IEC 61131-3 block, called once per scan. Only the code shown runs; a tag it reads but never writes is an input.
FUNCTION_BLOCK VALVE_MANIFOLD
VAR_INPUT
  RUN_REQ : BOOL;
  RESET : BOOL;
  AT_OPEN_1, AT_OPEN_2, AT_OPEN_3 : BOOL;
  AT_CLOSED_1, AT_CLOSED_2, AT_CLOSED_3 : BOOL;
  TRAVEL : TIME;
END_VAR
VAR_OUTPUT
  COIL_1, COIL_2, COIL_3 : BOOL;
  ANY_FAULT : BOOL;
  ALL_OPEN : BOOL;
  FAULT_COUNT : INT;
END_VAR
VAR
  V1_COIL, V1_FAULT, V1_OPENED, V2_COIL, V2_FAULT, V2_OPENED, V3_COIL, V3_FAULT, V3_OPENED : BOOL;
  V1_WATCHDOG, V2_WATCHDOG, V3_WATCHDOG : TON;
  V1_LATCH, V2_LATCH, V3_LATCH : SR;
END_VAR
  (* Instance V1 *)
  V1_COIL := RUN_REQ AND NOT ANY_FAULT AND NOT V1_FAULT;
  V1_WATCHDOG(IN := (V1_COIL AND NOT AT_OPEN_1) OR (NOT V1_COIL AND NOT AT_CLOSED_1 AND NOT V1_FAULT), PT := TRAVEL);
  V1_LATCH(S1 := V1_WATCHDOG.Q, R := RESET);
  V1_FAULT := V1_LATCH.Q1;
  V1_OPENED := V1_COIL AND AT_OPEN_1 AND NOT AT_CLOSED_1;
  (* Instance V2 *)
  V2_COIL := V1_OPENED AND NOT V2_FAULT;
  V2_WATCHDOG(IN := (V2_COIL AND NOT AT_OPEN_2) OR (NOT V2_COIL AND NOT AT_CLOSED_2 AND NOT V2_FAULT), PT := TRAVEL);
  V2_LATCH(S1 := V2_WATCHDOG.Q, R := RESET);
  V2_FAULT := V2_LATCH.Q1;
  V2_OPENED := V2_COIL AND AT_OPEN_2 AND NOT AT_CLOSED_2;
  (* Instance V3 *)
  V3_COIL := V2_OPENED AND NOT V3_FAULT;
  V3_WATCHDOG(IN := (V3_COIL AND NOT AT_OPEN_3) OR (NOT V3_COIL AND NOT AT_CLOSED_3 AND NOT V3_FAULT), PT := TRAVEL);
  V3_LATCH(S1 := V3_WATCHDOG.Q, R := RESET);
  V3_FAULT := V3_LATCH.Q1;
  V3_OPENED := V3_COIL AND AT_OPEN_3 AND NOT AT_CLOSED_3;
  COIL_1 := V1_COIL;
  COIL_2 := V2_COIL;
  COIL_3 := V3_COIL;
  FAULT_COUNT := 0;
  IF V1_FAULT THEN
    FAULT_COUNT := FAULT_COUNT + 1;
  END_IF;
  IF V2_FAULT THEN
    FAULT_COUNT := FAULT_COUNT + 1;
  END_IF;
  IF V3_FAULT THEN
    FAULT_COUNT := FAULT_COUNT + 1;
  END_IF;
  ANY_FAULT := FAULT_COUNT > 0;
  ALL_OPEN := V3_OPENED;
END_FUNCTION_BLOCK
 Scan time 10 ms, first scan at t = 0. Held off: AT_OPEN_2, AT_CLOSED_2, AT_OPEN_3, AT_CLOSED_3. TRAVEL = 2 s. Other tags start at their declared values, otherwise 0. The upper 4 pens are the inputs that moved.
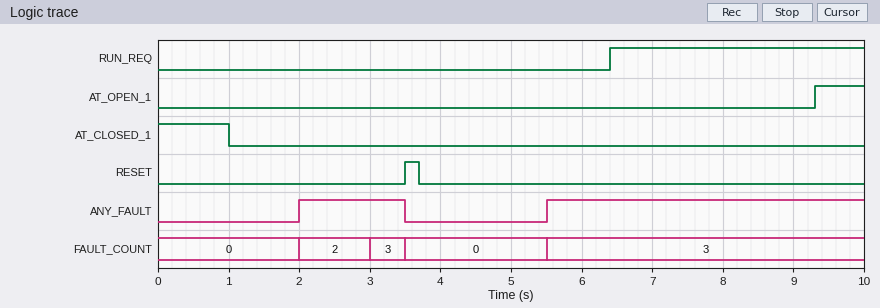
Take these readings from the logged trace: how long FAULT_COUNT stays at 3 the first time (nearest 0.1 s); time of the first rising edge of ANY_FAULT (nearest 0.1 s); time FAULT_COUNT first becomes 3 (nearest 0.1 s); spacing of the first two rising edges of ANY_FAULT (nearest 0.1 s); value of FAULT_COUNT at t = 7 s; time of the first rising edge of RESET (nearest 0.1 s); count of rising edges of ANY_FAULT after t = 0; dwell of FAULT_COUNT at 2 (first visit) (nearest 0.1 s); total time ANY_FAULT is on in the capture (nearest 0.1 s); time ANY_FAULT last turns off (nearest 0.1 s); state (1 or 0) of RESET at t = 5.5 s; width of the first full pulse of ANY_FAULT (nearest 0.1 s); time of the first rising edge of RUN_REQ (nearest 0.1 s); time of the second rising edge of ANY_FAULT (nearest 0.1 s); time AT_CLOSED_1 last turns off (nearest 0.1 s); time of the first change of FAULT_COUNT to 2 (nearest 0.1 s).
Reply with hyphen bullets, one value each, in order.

- 0.5 s
- 2.0 s
- 3.0 s
- 3.5 s
- 3
- 3.5 s
- 2
- 1.0 s
- 6.0 s
- 3.5 s
- 0
- 1.5 s
- 6.4 s
- 5.5 s
- 1.0 s
- 2.0 s
